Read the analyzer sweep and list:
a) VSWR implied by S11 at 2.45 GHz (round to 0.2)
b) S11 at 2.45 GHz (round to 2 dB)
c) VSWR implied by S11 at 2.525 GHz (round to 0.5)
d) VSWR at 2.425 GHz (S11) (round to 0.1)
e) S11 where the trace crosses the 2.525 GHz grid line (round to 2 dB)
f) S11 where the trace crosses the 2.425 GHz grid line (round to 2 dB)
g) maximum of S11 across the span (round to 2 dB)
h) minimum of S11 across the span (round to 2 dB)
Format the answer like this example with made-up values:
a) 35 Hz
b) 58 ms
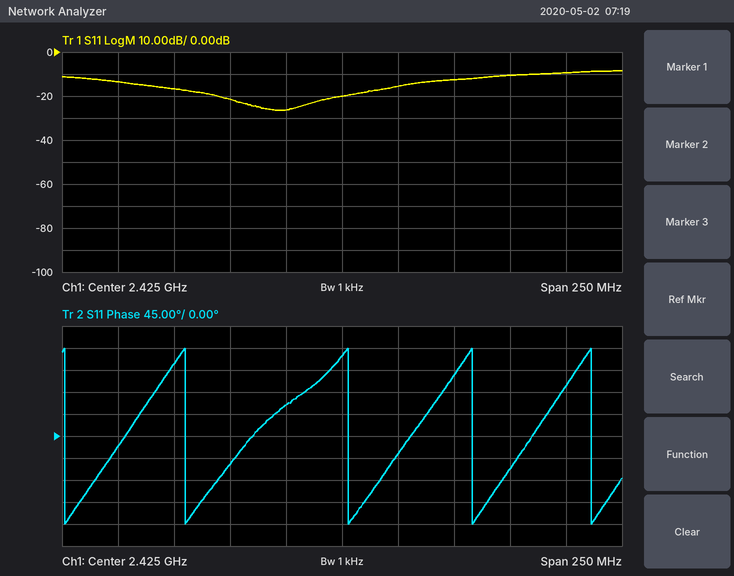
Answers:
a) 1.4
b) -16 dB
c) 2.0
d) 1.2
e) -10 dB
f) -20 dB
g) -8 dB
h) -26 dB
